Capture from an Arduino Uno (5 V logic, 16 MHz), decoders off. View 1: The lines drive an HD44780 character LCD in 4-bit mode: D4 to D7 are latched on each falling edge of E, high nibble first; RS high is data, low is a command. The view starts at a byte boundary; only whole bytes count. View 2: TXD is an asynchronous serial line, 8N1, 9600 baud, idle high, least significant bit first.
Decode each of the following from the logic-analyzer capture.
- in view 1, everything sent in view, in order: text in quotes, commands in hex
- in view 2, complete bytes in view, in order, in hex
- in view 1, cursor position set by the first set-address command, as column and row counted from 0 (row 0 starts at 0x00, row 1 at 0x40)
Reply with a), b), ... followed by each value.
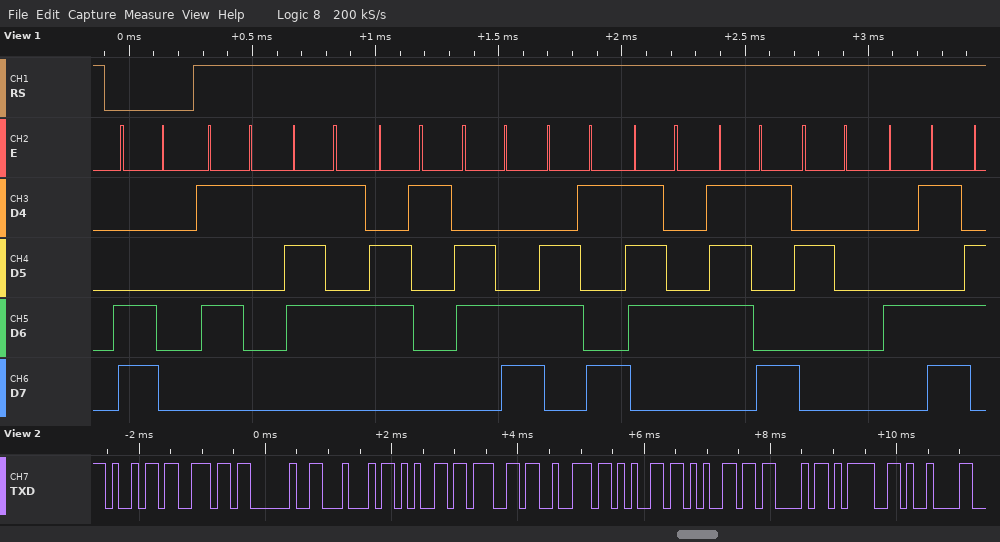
a) 0xC0 "Quality M"
b) 0x69 0x6E 0x20 0x44 0x65 0x67 0x72 0x65 0x65 0x43 0x3D 0x09
c) column 0, row 1
